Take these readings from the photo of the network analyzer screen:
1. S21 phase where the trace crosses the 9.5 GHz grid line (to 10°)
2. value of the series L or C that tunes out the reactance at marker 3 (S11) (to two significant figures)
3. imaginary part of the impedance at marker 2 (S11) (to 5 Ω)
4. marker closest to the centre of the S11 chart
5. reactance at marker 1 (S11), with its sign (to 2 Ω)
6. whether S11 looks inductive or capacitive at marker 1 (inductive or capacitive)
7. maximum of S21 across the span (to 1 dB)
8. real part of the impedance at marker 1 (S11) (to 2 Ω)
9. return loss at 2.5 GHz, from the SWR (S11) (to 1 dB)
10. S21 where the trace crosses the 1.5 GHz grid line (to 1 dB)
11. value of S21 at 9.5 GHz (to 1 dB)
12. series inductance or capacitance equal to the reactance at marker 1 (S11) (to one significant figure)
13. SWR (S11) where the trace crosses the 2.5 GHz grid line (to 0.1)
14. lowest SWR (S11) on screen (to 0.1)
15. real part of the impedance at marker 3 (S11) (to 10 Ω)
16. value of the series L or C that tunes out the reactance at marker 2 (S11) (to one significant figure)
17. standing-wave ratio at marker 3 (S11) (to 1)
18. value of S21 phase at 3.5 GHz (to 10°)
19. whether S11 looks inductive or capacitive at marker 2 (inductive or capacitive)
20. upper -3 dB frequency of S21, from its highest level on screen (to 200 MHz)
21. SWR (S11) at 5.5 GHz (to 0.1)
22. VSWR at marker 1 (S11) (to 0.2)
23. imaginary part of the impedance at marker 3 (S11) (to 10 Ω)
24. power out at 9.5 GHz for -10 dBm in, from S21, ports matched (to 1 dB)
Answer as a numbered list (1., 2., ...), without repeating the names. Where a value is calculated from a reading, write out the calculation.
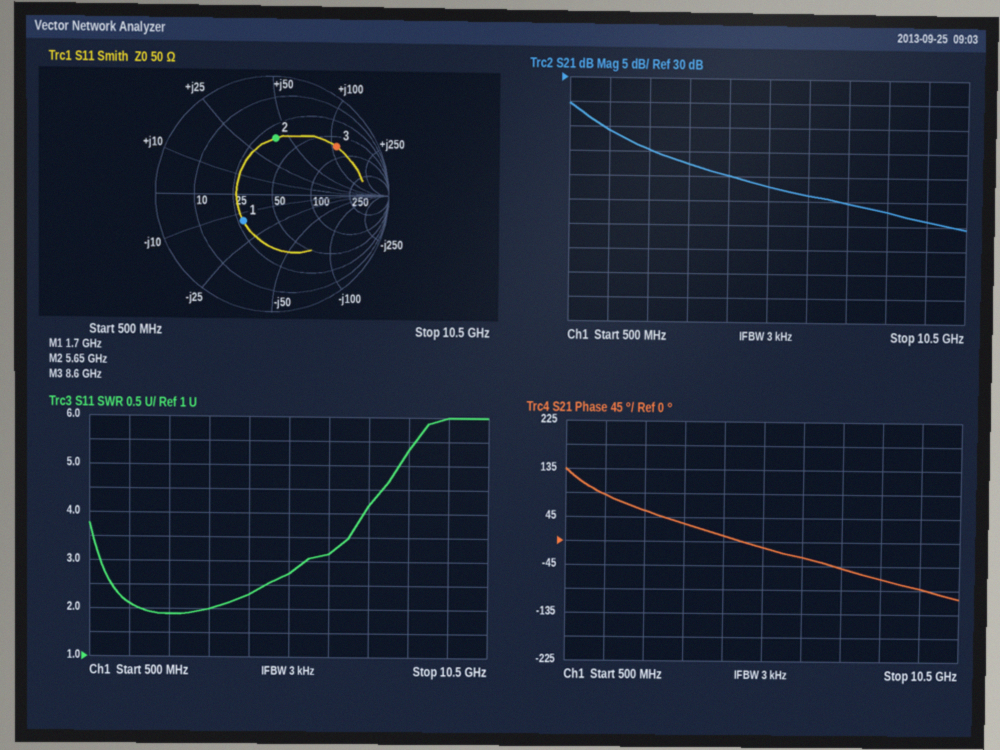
1. -90°
2. C = 1/(2π × 8.6 GHz × 110 Ω) ≈ 168 fF, so 170 fF to two significant figures
3. +40 Ω
4. marker 1
5. -14 Ω
6. capacitive
7. 25 dB
8. 28 Ω
9. −20 log10((1.9 − 1)/(1.9 + 1)) ≈ 10 dB
10. 19 dB
11. 1 dB
12. C = 1/(2π × 1.7 GHz × 14 Ω) ≈ 7 pF
13. 1.9
14. 1.9
15. 70 Ω
16. C = 1/(2π × 5.65 GHz × 40 Ω) ≈ 704 fF, so 700 fF to one significant figure
17. 5
18. 30°
19. inductive
20. 1.0 GHz
21. 2.7
22. 2.0
23. +110 Ω
24. -10 dBm + (1 dB) = -9 dBm
